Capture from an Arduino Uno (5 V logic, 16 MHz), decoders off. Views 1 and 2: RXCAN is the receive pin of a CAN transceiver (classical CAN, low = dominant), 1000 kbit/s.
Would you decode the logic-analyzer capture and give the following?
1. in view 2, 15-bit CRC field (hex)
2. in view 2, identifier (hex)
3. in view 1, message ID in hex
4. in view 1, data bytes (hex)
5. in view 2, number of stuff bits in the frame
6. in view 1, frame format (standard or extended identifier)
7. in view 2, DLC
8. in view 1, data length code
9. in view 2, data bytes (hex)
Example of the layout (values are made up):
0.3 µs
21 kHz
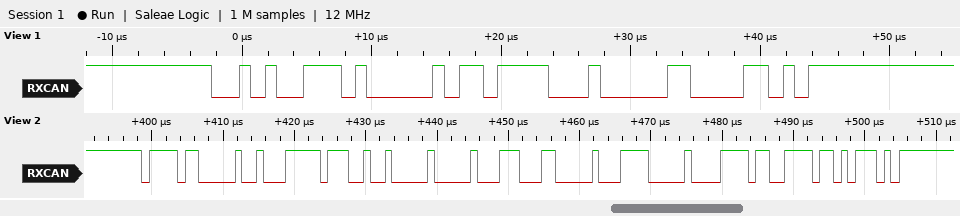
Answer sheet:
0x3DAE
0x7B0
0x29D
BC
6
standard
8
1
FF 24 00 1C 60 1E 00 F6
